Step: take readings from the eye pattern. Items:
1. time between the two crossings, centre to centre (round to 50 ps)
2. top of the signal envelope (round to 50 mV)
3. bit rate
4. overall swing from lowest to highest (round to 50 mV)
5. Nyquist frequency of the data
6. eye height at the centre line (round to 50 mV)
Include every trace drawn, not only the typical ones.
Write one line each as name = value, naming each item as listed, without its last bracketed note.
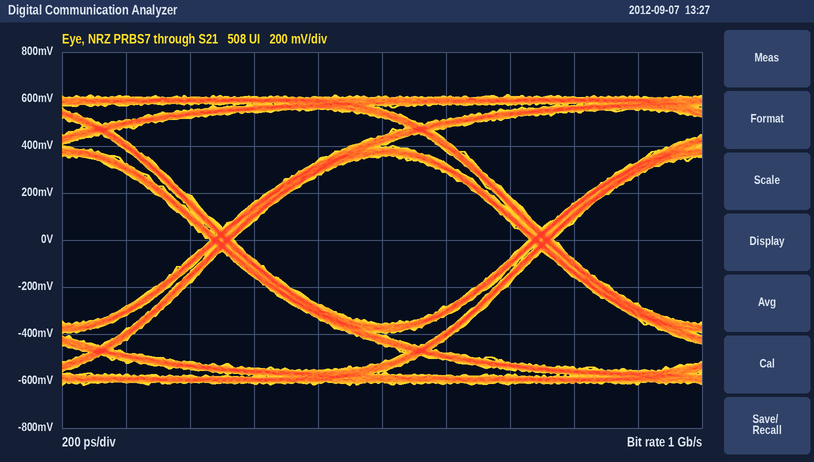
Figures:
time between the two crossings, centre to centre = 1.00 ns
top of the signal envelope = 600 mV
bit rate = 1 Gb/s
overall swing from lowest to highest = 1.25 V
Nyquist frequency of the data = 500 MHz
eye height at the centre line = 700 mV
